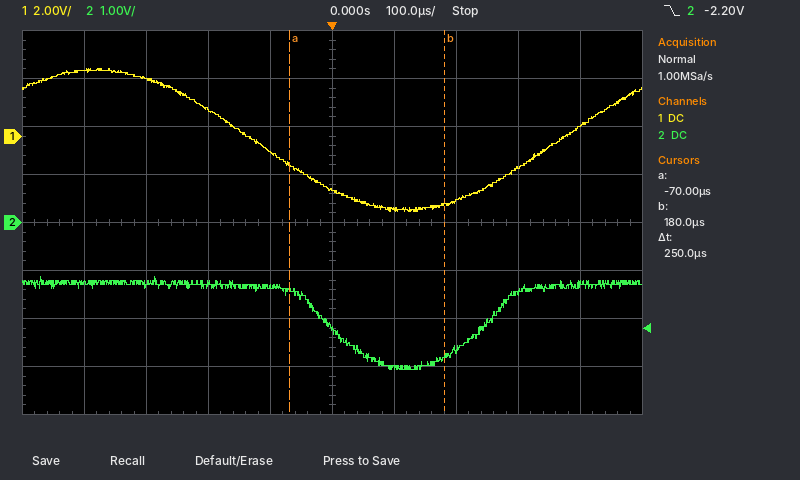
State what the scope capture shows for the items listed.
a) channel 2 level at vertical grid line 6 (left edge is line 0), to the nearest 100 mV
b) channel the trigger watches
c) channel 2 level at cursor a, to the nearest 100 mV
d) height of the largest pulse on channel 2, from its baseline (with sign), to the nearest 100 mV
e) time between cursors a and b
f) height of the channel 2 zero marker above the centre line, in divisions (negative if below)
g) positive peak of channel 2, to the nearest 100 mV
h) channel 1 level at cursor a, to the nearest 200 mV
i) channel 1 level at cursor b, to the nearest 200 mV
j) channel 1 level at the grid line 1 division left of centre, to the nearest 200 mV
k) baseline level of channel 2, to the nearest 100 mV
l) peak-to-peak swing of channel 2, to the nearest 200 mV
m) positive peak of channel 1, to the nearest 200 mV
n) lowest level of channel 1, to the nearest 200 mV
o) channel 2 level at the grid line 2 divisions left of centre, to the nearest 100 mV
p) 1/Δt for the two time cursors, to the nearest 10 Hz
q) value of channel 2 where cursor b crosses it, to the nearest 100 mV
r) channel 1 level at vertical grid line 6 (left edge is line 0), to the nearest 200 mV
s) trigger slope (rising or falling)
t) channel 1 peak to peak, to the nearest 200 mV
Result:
-3.0 V
channel 2
-1.4 V
-1.8 V
250 µs
0.0 div
-1.1 V
-1.2 V
-2.8 V
-600 mV
-1.3 V
2.0 V
2.8 V
-3.2 V
-1.3 V
4.00 kHz
-2.8 V
-3.0 V
falling
6.0 V
